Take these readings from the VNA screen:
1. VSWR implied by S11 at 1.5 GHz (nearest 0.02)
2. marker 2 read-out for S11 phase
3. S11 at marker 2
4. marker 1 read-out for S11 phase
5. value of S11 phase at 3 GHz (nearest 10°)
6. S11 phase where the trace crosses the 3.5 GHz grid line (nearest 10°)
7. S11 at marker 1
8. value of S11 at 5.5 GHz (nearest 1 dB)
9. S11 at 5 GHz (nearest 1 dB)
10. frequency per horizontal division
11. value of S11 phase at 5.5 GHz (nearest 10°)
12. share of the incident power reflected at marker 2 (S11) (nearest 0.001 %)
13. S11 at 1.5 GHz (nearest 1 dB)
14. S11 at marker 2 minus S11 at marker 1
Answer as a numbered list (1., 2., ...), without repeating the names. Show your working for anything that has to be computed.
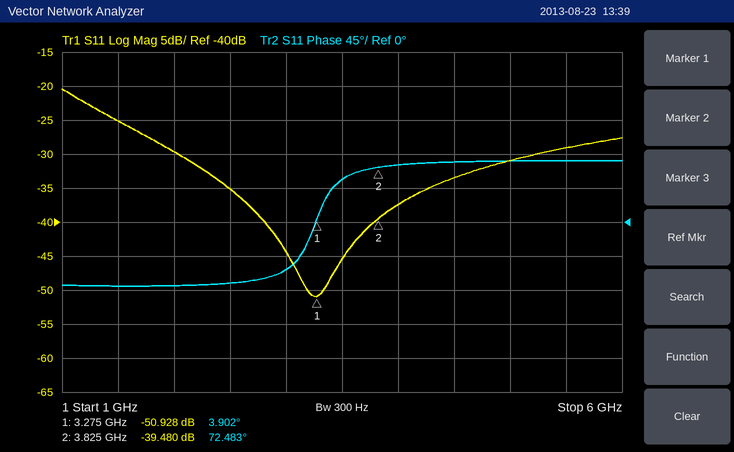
1. |Γ| = 10^(-25/20) = 0.0562; VSWR = (1 + 0.0562)/(1 − 0.0562) ≈ 1.12
2. 72.483°
3. -39.480 dB
4. 3.902°
5. -60°
6. 60°
7. -50.928 dB
8. -29 dB
9. -31 dB
10. 500 MHz
11. 80°
12. 10^(-39.48/10) ≈ 0.011 %
13. -25 dB
14. -39.48 − (-50.928) = 11.448 dB
